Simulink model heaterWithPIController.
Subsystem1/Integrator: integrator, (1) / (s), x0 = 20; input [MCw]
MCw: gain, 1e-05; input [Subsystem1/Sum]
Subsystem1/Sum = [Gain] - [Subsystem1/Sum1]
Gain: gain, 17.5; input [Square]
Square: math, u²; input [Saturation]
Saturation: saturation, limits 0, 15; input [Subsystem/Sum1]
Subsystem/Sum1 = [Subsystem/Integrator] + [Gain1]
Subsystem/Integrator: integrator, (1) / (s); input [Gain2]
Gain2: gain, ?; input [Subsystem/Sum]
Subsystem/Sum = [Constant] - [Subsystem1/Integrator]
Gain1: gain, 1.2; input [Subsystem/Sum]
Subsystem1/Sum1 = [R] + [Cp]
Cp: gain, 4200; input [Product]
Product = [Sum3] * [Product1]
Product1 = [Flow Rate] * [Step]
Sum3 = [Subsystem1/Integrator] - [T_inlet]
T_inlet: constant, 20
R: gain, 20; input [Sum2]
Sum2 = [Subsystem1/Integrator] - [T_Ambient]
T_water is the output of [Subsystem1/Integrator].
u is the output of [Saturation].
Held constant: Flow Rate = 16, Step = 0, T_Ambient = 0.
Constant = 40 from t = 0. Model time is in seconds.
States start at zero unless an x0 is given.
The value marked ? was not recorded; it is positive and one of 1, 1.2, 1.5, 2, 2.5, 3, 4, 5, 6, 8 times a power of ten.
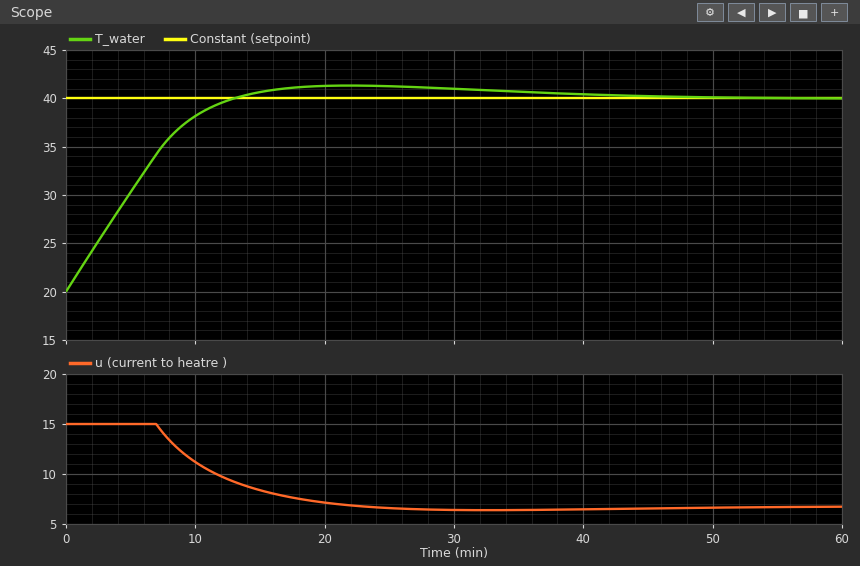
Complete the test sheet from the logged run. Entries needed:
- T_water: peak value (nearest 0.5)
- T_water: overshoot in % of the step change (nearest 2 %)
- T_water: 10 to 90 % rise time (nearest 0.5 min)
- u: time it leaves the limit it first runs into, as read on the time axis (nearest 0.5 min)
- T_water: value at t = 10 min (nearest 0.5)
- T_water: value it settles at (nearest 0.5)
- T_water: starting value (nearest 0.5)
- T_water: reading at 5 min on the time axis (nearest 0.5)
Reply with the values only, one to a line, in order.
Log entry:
41.5
6 %
9.0 min
7.0 min
38.0
40.0
20.0
30.5
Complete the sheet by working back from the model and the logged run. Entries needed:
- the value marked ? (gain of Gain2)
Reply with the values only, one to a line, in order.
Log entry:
0.0015
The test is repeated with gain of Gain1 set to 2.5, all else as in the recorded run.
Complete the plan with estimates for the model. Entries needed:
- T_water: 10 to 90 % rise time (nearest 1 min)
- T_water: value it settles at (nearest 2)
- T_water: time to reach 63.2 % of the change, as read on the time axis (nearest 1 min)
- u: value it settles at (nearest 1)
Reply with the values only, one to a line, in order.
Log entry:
8 min
40
6 min
7
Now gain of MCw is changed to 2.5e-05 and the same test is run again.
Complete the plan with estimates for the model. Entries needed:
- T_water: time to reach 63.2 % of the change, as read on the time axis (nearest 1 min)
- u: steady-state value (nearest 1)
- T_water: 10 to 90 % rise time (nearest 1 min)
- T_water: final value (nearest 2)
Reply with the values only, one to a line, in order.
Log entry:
3 min
7
8 min
40
